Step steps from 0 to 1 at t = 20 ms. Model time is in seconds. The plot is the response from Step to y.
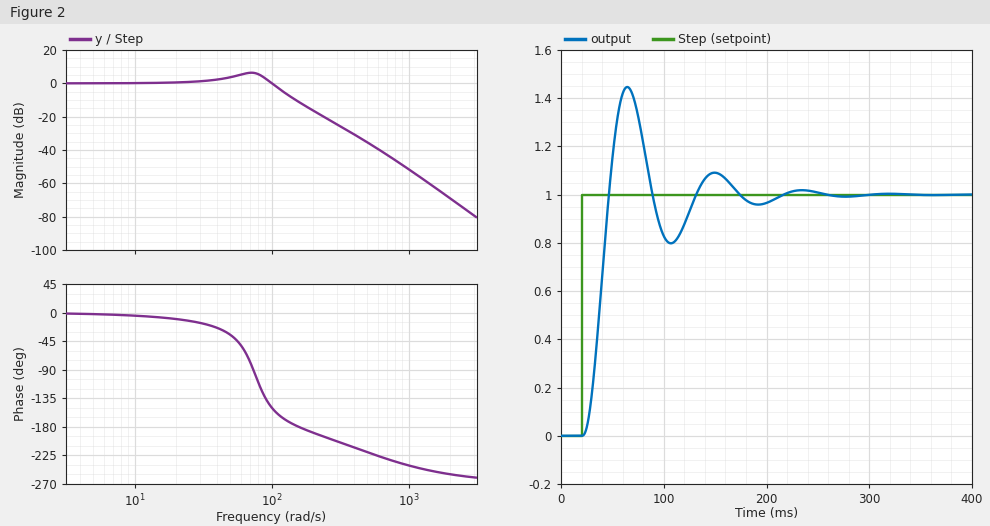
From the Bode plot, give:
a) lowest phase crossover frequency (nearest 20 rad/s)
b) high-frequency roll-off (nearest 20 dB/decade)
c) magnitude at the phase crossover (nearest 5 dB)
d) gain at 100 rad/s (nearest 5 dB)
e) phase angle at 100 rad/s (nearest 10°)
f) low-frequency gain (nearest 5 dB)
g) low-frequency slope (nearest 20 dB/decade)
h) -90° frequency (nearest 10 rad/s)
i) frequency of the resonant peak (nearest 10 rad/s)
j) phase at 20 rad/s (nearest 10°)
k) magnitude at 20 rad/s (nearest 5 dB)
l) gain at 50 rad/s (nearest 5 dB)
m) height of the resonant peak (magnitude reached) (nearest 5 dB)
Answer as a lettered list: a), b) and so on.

a) 160 rad/s
b) -60 dB/decade
c) -10 dB
d) 0 dB
e) -150°
f) 0 dB
g) 0 dB/decade
h) 70 rad/s
i) 70 rad/s
j) -10°
k) 0 dB
l) 5 dB
m) 5 dB
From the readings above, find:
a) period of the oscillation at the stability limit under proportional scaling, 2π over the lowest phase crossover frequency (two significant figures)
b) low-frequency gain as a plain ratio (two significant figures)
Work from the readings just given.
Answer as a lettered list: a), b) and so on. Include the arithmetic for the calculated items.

a) 2π / 160 = 0.039 s
b) 10^(0 / 20) = 1.0
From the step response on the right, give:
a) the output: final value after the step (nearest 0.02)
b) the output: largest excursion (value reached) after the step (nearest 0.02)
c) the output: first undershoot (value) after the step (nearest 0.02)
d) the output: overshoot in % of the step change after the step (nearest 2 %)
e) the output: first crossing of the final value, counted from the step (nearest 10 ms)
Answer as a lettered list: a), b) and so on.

a) 1.00
b) 1.44
c) 0.80
d) 44 %
e) 30 ms
